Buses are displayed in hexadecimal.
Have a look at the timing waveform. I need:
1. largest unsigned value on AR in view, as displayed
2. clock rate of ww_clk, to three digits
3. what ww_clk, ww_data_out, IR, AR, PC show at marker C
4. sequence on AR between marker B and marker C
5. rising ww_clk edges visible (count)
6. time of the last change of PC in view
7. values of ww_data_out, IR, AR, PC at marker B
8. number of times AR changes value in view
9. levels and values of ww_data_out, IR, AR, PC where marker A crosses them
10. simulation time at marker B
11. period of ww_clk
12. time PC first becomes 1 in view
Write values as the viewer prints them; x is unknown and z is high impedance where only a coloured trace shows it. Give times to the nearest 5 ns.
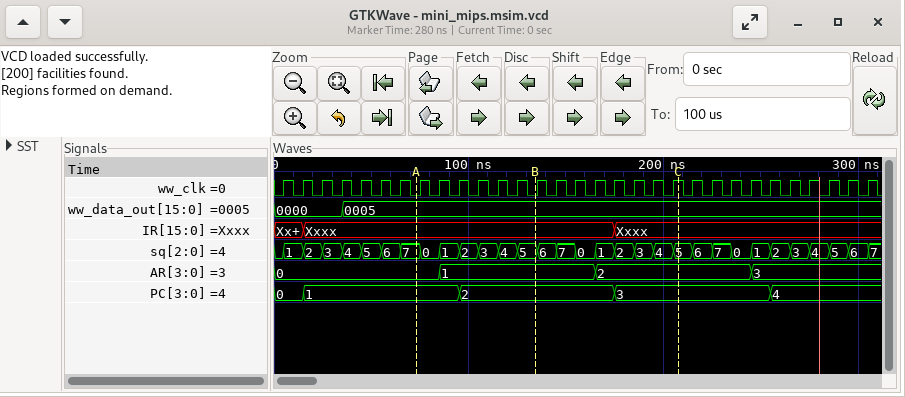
3
100 MHz
ww_clk=1, ww_data_out=0005, IR=Xxxx, AR=2, PC=3
1, 2
31
255 ns
ww_data_out=0005, IR=Xxxx, AR=1, PC=2
3
ww_data_out=0005, IR=Xxxx, AR=0, PC=1
135 ns
10 ns
15 ns
